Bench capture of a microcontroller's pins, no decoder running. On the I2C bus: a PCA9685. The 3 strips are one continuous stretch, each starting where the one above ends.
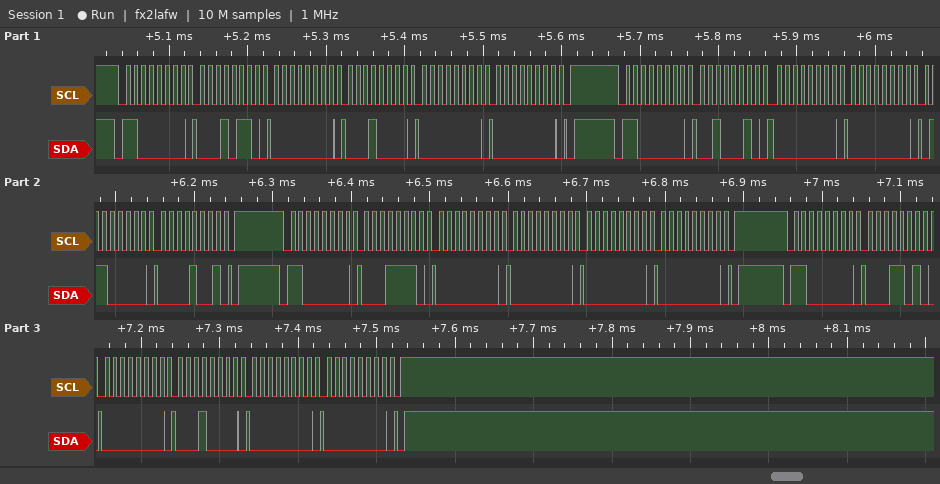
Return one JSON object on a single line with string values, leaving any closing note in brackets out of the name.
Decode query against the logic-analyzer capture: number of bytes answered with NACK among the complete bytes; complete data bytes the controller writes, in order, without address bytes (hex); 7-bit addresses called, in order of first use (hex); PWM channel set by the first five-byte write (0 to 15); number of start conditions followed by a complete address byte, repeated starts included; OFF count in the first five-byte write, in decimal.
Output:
{"number of bytes answered with NACK among the complete bytes": "0", "complete data bytes the controller writes, in order, without address bytes": "16 00 10 00 00 22 00 00 60 09 1E 00 00 00 00 1A 00 10 00 00", "7-bit addresses called, in order of first use": "0x60", "PWM channel set by the first five-byte write": "4", "number of start conditions followed by a complete address byte, repeated starts included": "4", "OFF count in the first five-byte write, in decimal": "0"}
